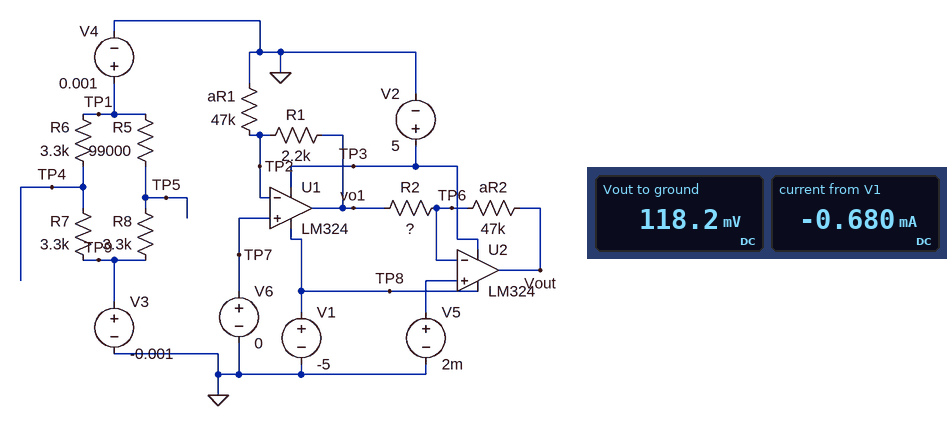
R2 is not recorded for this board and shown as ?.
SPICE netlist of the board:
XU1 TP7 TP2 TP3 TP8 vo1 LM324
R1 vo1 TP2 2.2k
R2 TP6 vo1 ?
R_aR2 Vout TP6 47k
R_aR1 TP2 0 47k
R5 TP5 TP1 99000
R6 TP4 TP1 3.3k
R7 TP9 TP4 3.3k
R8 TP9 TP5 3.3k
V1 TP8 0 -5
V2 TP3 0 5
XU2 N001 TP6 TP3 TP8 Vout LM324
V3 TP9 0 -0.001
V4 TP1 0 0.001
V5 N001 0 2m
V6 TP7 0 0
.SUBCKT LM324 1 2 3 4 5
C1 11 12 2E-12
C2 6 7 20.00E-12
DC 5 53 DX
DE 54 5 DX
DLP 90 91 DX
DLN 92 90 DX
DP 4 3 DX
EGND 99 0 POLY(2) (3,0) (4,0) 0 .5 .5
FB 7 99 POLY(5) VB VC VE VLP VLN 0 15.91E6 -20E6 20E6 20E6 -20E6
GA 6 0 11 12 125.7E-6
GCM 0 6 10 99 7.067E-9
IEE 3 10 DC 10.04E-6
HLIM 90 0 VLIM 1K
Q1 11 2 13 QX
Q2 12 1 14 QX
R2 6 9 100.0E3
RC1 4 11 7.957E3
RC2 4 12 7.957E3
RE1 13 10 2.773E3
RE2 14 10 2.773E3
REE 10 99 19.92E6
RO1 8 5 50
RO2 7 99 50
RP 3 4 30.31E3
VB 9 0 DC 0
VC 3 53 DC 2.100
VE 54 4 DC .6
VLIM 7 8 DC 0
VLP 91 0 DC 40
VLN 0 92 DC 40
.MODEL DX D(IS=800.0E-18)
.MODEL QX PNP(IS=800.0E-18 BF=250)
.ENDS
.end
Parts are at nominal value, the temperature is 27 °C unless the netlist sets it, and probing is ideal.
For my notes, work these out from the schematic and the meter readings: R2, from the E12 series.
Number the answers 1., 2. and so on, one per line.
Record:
1. 820 Ω
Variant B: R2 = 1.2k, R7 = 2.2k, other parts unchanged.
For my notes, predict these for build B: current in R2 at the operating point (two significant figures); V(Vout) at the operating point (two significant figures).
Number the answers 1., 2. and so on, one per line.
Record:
1. 1.7 µA
2. 81 mV
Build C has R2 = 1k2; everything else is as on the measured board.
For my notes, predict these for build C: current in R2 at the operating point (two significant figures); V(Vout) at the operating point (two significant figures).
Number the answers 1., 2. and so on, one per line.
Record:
1. 1.7 µA
2. 81 mV
